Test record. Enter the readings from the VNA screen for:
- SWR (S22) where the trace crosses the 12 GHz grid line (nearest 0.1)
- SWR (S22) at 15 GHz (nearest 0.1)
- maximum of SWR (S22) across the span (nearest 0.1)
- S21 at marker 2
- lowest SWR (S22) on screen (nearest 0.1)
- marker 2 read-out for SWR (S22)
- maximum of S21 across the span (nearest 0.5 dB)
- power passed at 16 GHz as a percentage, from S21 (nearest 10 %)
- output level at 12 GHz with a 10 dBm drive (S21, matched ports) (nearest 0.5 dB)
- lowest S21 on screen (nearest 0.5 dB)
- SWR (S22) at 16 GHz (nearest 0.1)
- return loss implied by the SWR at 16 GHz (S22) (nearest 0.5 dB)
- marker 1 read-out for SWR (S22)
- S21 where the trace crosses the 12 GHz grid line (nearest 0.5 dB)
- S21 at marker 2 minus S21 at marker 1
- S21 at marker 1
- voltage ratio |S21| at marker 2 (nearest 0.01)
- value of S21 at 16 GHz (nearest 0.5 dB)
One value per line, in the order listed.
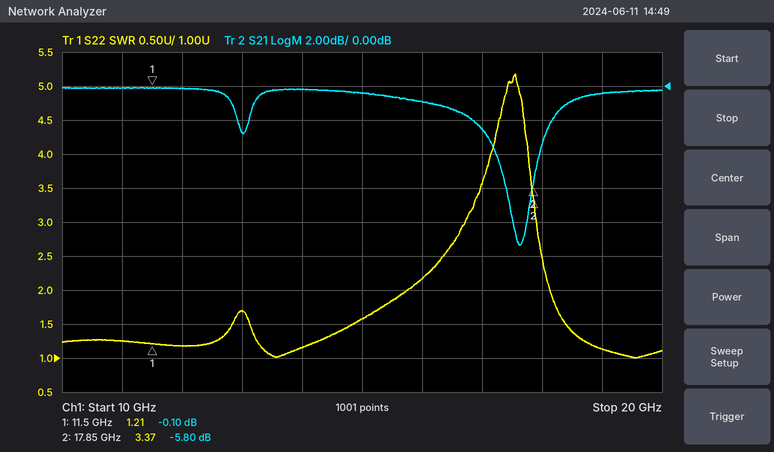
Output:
1.2
1.6
5.2
-5.80 dB
1.0
3.37
0.0 dB
80 %
10.0 dBm
-9.5 dB
2.2
8.5 dB
1.21
0.0 dB
-5.70 dB
-0.10 dB
0.51
-1.0 dB
